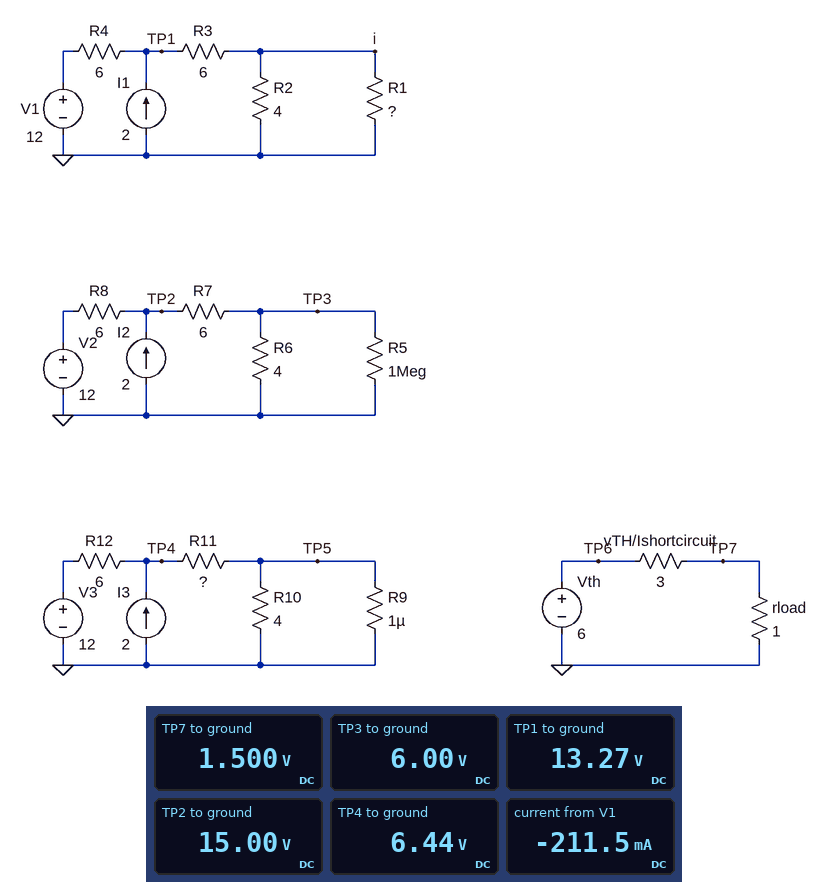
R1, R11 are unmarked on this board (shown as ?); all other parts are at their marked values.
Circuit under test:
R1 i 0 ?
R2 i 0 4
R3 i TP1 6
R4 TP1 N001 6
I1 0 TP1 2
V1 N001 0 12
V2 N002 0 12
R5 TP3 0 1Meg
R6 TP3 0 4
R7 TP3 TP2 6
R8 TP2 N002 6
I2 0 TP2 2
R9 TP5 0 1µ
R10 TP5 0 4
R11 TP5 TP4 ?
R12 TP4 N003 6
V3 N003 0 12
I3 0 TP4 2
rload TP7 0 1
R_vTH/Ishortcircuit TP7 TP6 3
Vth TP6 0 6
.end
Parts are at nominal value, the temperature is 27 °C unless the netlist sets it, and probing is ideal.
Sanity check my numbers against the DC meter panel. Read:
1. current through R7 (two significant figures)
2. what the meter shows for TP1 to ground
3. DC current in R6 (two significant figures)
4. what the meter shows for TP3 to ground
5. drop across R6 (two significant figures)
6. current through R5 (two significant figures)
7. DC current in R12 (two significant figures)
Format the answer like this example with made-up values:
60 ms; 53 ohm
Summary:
1.5 A; 13.27 V; 1.5 A; 6.00 V; 6.0 V; 6.0 µA; 930 mA
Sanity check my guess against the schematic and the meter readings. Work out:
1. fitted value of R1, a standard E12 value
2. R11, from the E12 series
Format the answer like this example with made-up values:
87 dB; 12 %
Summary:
2.2 Ω; 2.2 Ω
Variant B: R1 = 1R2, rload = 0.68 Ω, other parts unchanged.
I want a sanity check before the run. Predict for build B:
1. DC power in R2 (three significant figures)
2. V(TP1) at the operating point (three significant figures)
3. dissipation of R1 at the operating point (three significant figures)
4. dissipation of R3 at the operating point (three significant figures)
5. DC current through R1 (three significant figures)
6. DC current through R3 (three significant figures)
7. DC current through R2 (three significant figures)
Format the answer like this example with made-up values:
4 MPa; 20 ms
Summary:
735 mW; 12.9 V; 2.45 W; 20.7 W; 1.43 A; 1.86 A; 429 mA
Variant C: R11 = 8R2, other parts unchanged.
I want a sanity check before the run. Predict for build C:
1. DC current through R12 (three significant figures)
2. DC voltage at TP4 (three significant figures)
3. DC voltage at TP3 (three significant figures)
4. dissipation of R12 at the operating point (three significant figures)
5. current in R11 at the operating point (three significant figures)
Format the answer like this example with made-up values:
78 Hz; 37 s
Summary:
310 mA; 13.9 V; 6.00 V; 576 mW; 1.69 A
